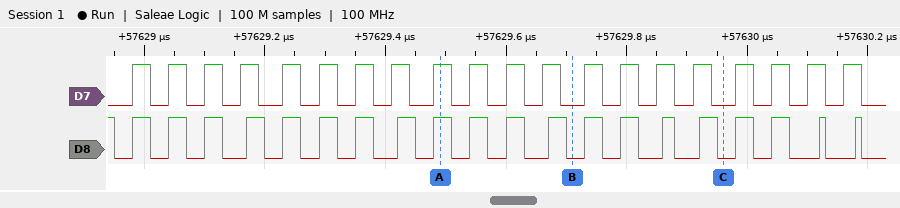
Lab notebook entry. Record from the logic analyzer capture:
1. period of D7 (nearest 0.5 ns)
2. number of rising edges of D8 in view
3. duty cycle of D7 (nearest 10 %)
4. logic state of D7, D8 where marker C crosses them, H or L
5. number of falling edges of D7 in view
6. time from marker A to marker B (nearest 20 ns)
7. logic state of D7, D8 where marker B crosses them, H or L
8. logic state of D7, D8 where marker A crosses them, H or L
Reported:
62 ns
20
50 %
D7=L, D8=L
20
220 ns
D7=L, D8=L
D7=H, D8=H
